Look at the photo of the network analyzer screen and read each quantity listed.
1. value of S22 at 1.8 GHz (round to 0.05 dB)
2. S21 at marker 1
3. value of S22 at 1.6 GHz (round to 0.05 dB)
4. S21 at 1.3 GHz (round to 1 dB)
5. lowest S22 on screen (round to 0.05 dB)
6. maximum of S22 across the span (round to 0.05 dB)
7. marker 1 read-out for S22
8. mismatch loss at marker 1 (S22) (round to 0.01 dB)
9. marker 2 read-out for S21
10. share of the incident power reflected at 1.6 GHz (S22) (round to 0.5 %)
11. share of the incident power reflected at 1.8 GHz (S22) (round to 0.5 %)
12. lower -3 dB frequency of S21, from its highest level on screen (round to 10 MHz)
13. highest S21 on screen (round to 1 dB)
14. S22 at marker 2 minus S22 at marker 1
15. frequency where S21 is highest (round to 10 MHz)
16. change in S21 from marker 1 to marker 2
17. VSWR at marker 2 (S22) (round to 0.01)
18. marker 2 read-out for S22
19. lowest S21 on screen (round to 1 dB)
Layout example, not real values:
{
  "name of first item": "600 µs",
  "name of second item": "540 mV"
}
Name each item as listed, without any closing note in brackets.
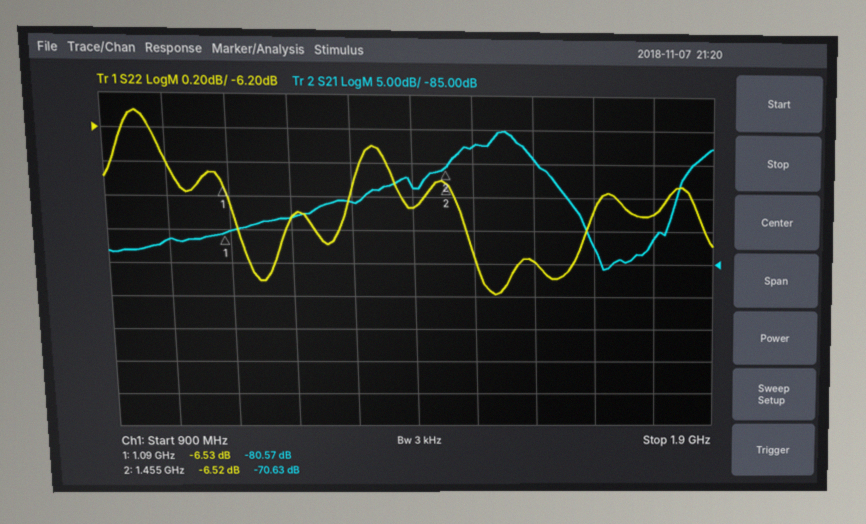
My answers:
{
  "value of S22 at 1.8 GHz": "-6.70 dB",
  "S21 at marker 1": "-80.57 dB",
  "value of S22 at 1.6 GHz": "-7.00 dB",
  "S21 at 1.3 GHz": "-76 dB",
  "lowest S22 on screen": "-7.20 dB",
  "maximum of S22 across the span": "-6.10 dB",
  "marker 1 read-out for S22": "-6.53 dB",
  "mismatch loss at marker 1 (S22)": "1.09 dB",
  "marker 2 read-out for S21": "-70.63 dB",
  "share of the incident power reflected at 1.6 GHz (S22)": "20.0 %",
  "share of the incident power reflected at 1.8 GHz (S22)": "21.5 %",
  "lower -3 dB frequency of S21, from its highest level on screen": "1.48 GHz",
  "highest S21 on screen": "-65 dB",
  "S22 at marker 2 minus S22 at marker 1": "0.01 dB",
  "frequency where S21 is highest": "1.55 GHz",
  "change in S21 from marker 1 to marker 2": "9.94 dB",
  "VSWR at marker 2 (S22)": "2.79",
  "marker 2 read-out for S22": "-6.52 dB",
  "lowest S21 on screen": "-86 dB"
}
